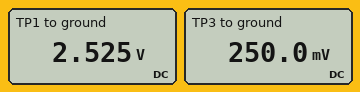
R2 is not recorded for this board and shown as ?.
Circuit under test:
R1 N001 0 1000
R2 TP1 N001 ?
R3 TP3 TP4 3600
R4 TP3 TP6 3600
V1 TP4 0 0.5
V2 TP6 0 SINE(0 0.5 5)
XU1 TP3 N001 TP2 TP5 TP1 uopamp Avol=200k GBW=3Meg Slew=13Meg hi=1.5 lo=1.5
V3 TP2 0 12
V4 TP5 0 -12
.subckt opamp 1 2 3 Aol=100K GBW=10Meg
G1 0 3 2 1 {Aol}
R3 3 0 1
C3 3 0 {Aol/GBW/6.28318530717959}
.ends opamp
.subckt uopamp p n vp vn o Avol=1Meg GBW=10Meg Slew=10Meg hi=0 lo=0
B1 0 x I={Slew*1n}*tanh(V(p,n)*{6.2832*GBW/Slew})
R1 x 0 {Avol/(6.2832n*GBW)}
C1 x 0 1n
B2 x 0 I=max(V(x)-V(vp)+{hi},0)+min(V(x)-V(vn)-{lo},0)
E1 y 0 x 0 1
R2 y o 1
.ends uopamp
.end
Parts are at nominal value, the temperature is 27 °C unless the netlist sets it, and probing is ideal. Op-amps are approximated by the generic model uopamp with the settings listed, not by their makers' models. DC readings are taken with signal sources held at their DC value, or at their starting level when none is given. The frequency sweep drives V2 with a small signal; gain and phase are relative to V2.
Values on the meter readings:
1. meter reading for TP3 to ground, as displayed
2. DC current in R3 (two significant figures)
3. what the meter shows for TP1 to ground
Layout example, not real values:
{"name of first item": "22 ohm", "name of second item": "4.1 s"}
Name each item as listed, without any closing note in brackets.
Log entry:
{"meter reading for TP3 to ground, as displayed": "250.0 mV", "DC current in R3": "69 µA", "what the meter shows for TP1 to ground": "2.525 V"}
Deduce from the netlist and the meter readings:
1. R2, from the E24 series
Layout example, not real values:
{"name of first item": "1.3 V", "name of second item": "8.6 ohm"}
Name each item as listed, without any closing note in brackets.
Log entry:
{"R2, from the E24 series": "9.1 kΩ"}
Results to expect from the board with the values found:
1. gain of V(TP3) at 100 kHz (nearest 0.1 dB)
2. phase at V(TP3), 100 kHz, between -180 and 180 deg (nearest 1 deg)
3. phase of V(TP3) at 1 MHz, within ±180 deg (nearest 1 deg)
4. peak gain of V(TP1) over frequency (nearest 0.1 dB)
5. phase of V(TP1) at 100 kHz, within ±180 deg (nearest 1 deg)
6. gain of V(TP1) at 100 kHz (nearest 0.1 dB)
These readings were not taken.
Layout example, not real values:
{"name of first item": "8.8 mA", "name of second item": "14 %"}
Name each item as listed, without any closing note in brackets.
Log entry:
{"gain of V(TP3) at 100 kHz": "-6.0 dB", "phase at V(TP3), 100 kHz, between -180 and 180 deg": "0 deg", "phase of V(TP3) at 1 MHz, within ±180 deg": "0 deg", "peak gain of V(TP1) over frequency": "14.1 dB", "phase of V(TP1) at 100 kHz, within ±180 deg": "-19 deg", "gain of V(TP1) at 100 kHz": "13.6 dB"}
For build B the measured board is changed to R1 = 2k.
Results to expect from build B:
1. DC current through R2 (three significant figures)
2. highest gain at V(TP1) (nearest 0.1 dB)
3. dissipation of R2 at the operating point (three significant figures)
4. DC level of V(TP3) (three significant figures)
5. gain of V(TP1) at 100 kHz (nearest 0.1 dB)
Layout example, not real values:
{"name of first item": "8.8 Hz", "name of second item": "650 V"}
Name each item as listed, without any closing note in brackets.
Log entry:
{"DC current through R2": "125 µA", "highest gain at V(TP1)": "8.9 dB", "dissipation of R2 at the operating point": "142 µW", "DC level of V(TP3)": "250 mV", "gain of V(TP1) at 100 kHz": "8.7 dB"}
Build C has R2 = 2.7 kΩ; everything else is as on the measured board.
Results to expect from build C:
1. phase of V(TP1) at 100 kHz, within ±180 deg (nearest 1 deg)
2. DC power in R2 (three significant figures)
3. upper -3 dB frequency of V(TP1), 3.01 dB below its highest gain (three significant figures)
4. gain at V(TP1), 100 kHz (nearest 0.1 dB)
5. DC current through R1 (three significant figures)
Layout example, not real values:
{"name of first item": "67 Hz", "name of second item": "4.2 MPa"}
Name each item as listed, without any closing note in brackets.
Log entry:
{"phase of V(TP1) at 100 kHz, within ±180 deg": "-7 deg", "DC power in R2": "169 µW", "upper -3 dB frequency of V(TP1), 3.01 dB below its highest gain": "811 kHz", "gain at V(TP1), 100 kHz": "5.3 dB", "DC current through R1": "250 µA"}
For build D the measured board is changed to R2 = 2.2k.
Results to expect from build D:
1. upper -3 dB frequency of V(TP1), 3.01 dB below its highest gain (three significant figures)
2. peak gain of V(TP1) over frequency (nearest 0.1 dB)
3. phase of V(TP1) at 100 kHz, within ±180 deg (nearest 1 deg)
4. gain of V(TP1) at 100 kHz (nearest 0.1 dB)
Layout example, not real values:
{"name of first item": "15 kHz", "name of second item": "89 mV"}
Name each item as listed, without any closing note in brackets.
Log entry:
{"upper -3 dB frequency of V(TP1), 3.01 dB below its highest gain": "937 kHz", "peak gain of V(TP1) over frequency": "4.1 dB", "phase of V(TP1) at 100 kHz, within ±180 deg": "-6 deg", "gain of V(TP1) at 100 kHz": "4.0 dB"}
